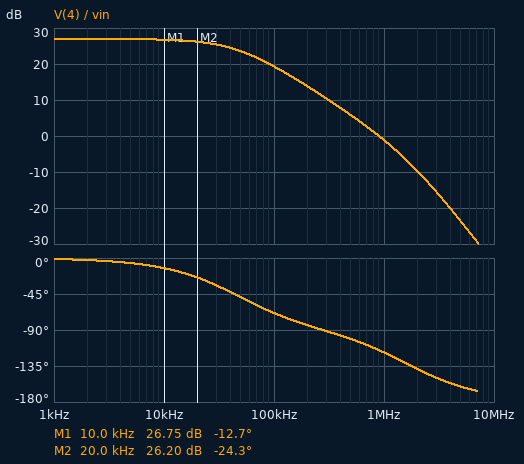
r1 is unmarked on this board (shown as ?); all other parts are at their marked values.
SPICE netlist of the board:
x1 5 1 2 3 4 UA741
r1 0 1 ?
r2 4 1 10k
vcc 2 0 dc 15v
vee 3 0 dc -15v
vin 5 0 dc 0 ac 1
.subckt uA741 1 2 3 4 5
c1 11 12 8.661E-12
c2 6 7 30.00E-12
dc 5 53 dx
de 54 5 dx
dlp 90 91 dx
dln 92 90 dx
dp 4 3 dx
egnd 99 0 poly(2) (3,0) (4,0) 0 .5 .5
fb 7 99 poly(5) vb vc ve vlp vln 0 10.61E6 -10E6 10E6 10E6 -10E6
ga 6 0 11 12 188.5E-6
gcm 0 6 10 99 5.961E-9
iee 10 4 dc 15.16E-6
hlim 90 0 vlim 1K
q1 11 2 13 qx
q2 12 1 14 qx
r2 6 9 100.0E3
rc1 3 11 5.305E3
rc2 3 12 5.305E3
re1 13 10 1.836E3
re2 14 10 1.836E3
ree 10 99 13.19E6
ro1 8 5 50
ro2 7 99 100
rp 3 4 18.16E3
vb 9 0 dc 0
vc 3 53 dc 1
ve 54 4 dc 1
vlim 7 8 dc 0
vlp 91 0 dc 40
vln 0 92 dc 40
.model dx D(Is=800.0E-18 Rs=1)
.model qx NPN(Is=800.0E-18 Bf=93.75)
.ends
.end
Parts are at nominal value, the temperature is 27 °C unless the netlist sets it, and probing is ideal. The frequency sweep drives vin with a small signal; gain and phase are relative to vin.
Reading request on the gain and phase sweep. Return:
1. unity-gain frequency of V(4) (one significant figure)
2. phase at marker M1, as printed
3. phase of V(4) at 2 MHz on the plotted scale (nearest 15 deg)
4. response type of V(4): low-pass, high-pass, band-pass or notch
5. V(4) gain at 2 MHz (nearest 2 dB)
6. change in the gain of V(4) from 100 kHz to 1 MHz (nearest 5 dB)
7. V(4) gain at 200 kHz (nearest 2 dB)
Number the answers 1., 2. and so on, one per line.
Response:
1. 900 kHz
2. -12.7 deg
3. -135 deg
4. low-pass
5. -10 dB
6. -20 dB
7. 14 dB
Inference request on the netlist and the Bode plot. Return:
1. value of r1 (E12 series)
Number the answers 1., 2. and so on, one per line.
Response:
1. 470 Ω
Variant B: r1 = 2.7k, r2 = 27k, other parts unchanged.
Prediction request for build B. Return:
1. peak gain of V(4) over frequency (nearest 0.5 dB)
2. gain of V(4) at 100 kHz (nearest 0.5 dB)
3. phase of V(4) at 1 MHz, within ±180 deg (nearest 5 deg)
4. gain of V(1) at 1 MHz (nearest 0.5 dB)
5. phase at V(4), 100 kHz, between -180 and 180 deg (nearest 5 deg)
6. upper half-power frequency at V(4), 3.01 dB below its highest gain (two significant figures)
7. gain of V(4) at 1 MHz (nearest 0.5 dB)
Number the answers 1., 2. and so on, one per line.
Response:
1. 21.0 dB
2. 17.5 dB
3. -115 deg
4. -22.0 dB
5. -50 deg
6. 95 kHz
7. -1.0 dB
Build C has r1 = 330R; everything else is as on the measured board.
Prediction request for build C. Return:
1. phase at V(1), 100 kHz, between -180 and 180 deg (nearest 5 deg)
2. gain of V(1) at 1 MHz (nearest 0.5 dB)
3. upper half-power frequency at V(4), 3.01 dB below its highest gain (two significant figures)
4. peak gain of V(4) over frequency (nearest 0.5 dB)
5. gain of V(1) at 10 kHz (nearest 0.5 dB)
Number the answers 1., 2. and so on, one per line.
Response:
1. -75 deg
2. -31.0 dB
3. 32 kHz
4. 30.0 dB
5. -0.5 dB
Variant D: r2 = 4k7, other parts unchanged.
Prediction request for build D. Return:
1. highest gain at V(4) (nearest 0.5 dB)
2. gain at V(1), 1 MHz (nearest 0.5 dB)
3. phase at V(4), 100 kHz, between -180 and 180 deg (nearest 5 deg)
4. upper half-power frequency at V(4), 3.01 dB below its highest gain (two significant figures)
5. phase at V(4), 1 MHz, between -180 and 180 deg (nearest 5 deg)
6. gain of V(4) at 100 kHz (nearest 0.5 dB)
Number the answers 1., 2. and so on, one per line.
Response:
1. 21.0 dB
2. -22.0 dB
3. -50 deg
4. 95 kHz
5. -115 deg
6. 17.5 dB
